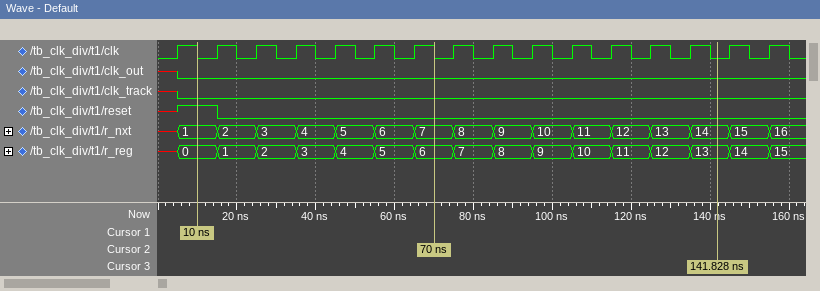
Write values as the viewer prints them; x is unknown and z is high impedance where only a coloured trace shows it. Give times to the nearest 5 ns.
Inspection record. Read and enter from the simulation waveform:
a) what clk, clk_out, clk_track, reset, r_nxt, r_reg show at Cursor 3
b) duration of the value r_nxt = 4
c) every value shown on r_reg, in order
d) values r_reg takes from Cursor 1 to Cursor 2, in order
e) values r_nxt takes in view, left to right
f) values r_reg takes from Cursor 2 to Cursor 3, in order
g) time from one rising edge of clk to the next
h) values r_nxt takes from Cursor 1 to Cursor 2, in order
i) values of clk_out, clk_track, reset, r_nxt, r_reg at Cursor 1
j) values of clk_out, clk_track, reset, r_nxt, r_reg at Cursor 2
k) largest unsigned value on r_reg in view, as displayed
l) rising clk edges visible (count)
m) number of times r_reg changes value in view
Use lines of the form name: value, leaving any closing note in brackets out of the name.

what clk, clk_out, clk_track, reset, r_nxt, r_reg show at Cursor 3: clk=0, clk_out=0, clk_track=0, reset=0, r_nxt=14, r_reg=13
duration of the value r_nxt = 4: 10 ns
every value shown on r_reg, in order: x, 0, 1, 2, 3, 4, 5, 6, 7, 8, 9, 10, 11, 12, 13, 14, 15
values r_reg takes from Cursor 1 to Cursor 2, in order: 0, 1, 2, 3, 4, 5, 6
values r_nxt takes in view, left to right: x, 1, 2, 3, 4, 5, 6, 7, 8, 9, 10, 11, 12, 13, 14, 15, 16
values r_reg takes from Cursor 2 to Cursor 3, in order: 6, 7, 8, 9, 10, 11, 12, 13
time from one rising edge of clk to the next: 10 ns
values r_nxt takes from Cursor 1 to Cursor 2, in order: 1, 2, 3, 4, 5, 6, 7
values of clk_out, clk_track, reset, r_nxt, r_reg at Cursor 1: clk_out=0, clk_track=0, reset=1, r_nxt=1, r_reg=0
values of clk_out, clk_track, reset, r_nxt, r_reg at Cursor 2: clk_out=0, clk_track=0, reset=0, r_nxt=7, r_reg=6
largest unsigned value on r_reg in view, as displayed: 15
rising clk edges visible: 16
number of times r_reg changes value in view: 16
